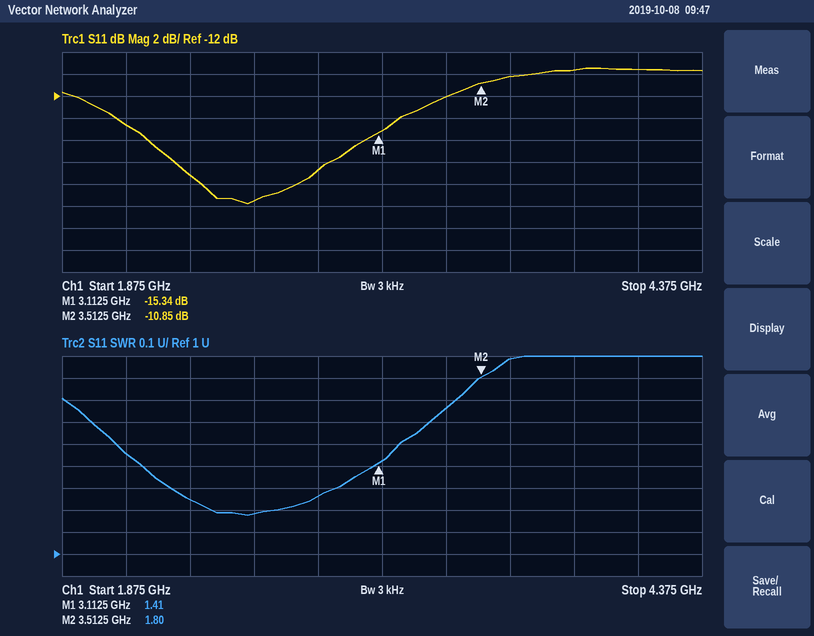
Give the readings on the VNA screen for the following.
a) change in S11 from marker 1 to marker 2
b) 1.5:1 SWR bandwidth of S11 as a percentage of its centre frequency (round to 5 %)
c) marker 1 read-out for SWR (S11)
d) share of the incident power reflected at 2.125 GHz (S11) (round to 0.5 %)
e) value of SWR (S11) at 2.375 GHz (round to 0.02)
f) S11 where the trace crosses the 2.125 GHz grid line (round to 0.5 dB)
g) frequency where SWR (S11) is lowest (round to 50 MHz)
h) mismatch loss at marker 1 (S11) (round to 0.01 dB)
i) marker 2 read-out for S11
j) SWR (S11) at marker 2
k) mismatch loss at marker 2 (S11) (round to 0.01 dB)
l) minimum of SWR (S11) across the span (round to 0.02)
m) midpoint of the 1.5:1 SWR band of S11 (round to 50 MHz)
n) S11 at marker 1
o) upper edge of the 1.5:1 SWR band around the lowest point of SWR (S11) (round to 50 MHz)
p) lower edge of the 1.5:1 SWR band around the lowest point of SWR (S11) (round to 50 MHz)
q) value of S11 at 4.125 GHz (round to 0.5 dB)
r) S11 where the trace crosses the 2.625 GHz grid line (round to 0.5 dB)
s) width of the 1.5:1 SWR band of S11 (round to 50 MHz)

4.49 dB
40 %
1.41
3.5 %
1.24
-14.5 dB
2.60 GHz
0.13 dB
-10.85 dB
1.80
0.37 dB
1.18
2.65 GHz
-15.34 dB
3.20 GHz
2.10 GHz
-9.5 dB
-21.5 dB
1.10 GHz
